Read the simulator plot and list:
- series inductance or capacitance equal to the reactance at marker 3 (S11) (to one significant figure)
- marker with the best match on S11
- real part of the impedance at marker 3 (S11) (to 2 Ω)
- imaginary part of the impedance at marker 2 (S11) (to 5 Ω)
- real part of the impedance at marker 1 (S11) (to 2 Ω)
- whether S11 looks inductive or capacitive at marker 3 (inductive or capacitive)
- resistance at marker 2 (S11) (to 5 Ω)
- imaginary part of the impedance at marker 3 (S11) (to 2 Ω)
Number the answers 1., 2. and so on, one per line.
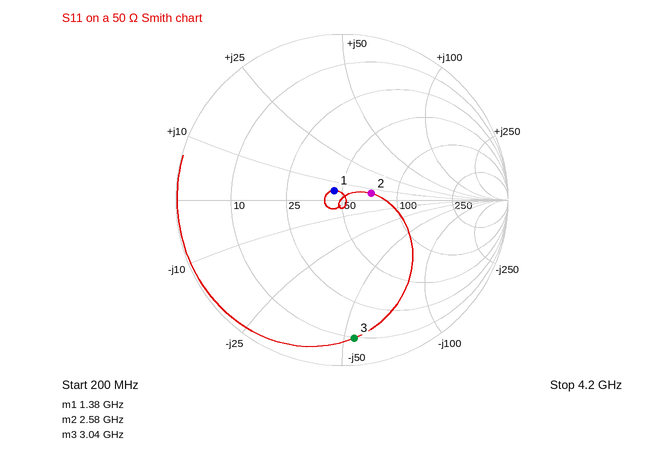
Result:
1. 1.0 pF
2. marker 1
3. 10 Ω
4. +5 Ω
5. 46 Ω
6. capacitive
7. 70 Ω
8. -54 Ω
